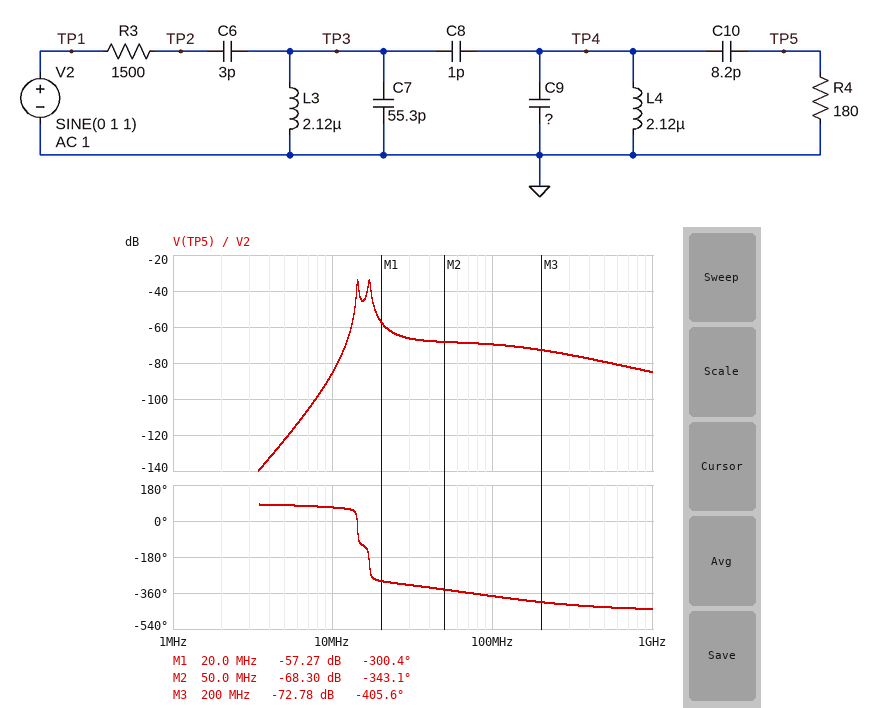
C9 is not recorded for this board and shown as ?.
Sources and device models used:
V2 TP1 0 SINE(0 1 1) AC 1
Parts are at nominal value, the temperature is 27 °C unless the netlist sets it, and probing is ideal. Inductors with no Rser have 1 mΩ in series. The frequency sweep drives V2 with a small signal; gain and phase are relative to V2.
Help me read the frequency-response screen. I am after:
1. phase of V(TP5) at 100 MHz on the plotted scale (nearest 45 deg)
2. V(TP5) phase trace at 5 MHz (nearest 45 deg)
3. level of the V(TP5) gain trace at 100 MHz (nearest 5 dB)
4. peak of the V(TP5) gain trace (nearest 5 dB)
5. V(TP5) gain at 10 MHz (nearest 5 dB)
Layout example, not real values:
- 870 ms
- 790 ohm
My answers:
- -360 deg
- 90 deg
- -70 dB
- -35 dB
- -85 dB
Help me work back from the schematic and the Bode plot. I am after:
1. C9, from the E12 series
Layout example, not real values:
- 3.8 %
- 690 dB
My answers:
- 33 pF
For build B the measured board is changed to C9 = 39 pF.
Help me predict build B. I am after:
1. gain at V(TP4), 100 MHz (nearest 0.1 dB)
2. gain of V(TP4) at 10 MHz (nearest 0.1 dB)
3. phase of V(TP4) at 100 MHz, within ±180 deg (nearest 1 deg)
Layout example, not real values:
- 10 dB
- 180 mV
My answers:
- -67.6 dB
- -63.5 dB
- -64 deg
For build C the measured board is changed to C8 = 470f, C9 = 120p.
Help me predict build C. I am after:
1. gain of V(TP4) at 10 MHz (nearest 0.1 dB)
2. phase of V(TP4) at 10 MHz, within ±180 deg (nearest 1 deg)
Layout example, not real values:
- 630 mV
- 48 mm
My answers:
- -52.3 dB
- 168 deg
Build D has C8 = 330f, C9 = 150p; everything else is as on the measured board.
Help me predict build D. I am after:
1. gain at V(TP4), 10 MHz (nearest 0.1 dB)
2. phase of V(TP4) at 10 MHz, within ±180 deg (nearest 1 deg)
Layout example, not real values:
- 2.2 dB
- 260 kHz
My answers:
- -68.0 dB
- 165 deg
